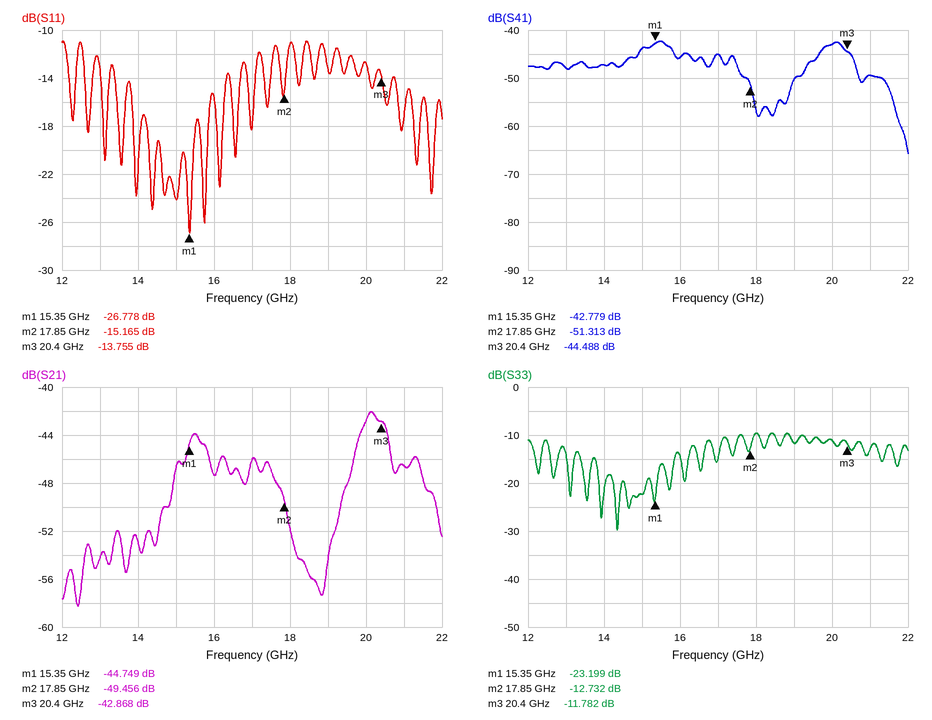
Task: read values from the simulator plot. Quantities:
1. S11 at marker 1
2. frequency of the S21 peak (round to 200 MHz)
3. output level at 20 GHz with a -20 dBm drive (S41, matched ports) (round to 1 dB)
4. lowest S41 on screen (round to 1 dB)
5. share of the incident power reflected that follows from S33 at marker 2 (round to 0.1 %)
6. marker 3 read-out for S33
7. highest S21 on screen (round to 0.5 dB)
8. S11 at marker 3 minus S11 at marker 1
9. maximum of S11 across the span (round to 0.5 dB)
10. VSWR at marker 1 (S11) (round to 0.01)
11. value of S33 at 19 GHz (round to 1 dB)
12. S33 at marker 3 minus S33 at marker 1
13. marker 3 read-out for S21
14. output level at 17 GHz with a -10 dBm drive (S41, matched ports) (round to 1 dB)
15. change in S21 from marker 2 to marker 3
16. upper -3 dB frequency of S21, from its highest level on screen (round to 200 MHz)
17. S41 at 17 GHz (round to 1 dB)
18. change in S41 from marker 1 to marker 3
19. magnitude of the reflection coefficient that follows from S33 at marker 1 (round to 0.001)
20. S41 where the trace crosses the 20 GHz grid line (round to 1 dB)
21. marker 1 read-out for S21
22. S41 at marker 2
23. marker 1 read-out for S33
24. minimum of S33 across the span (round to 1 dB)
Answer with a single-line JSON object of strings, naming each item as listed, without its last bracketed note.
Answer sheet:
{"S11 at marker 1": "-26.778 dB", "frequency of the S21 peak": "20.2 GHz", "output level at 20 GHz with a -20 dBm drive (S41, matched ports)": "-63 dBm", "lowest S41 on screen": "-66 dB", "share of the incident power reflected that follows from S33 at marker 2": "5.3 %", "marker 3 read-out for S33": "-11.782 dB", "highest S21 on screen": "-42.0 dB", "S11 at marker 3 minus S11 at marker 1": "13.023 dB", "maximum of S11 across the span": "-11.0 dB", "VSWR at marker 1 (S11)": "1.10", "value of S33 at 19 GHz": "-12 dB", "S33 at marker 3 minus S33 at marker 1": "11.417 dB", "marker 3 read-out for S21": "-42.868 dB", "output level at 17 GHz with a -10 dBm drive (S41, matched ports)": "-55 dBm", "change in S21 from marker 2 to marker 3": "6.588 dB", "upper -3 dB frequency of S21, from its highest level on screen": "20.6 GHz", "S41 at 17 GHz": "-45 dB", "change in S41 from marker 1 to marker 3": "-1.709 dB", "magnitude of the reflection coefficient that follows from S33 at marker 1": "0.069", "S41 where the trace crosses the 20 GHz grid line": "-43 dB", "marker 1 read-out for S21": "-44.749 dB", "S41 at marker 2": "-51.313 dB", "marker 1 read-out for S33": "-23.199 dB", "minimum of S33 across the span": "-30 dB"}
